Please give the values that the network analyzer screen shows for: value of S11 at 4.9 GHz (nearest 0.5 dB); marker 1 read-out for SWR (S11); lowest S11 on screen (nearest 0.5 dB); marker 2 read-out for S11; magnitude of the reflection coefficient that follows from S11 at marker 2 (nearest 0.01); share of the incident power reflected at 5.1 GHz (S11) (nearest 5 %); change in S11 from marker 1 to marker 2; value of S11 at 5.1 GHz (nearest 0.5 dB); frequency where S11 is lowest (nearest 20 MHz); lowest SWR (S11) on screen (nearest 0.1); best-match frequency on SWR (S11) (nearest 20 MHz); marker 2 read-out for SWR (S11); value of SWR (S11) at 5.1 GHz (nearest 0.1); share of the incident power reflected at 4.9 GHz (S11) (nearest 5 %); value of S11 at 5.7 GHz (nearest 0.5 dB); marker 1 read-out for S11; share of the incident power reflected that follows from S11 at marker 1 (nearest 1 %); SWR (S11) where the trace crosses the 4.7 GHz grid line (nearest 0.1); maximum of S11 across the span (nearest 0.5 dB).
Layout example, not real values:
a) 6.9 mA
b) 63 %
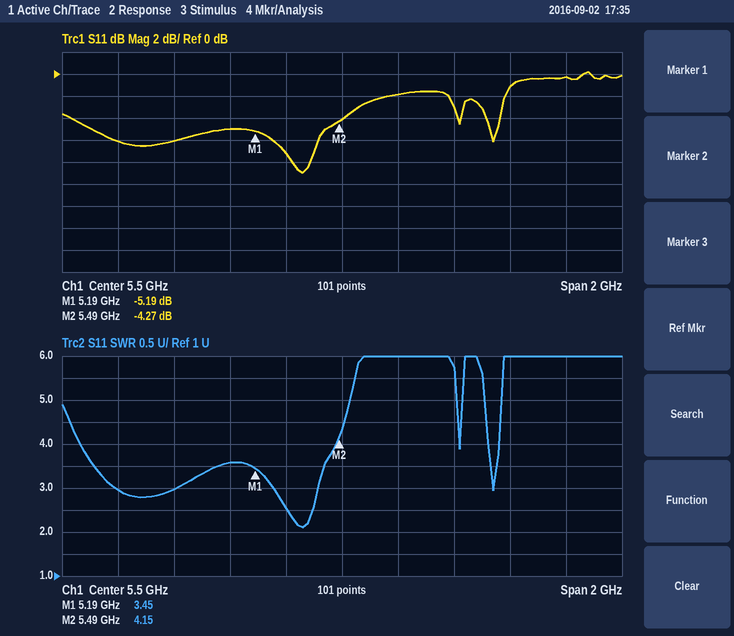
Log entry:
a) -6.0 dB
b) 3.45
c) -9.0 dB
d) -4.27 dB
e) 0.61
f) 30 %
g) 0.92 dB
h) -5.0 dB
i) 5.36 GHz
j) 2.1
k) 5.36 GHz
l) 4.15
m) 3.6
n) 25 %
o) -2.0 dB
p) -5.19 dB
q) 30 %
r) 3.0
s) 0.0 dB
